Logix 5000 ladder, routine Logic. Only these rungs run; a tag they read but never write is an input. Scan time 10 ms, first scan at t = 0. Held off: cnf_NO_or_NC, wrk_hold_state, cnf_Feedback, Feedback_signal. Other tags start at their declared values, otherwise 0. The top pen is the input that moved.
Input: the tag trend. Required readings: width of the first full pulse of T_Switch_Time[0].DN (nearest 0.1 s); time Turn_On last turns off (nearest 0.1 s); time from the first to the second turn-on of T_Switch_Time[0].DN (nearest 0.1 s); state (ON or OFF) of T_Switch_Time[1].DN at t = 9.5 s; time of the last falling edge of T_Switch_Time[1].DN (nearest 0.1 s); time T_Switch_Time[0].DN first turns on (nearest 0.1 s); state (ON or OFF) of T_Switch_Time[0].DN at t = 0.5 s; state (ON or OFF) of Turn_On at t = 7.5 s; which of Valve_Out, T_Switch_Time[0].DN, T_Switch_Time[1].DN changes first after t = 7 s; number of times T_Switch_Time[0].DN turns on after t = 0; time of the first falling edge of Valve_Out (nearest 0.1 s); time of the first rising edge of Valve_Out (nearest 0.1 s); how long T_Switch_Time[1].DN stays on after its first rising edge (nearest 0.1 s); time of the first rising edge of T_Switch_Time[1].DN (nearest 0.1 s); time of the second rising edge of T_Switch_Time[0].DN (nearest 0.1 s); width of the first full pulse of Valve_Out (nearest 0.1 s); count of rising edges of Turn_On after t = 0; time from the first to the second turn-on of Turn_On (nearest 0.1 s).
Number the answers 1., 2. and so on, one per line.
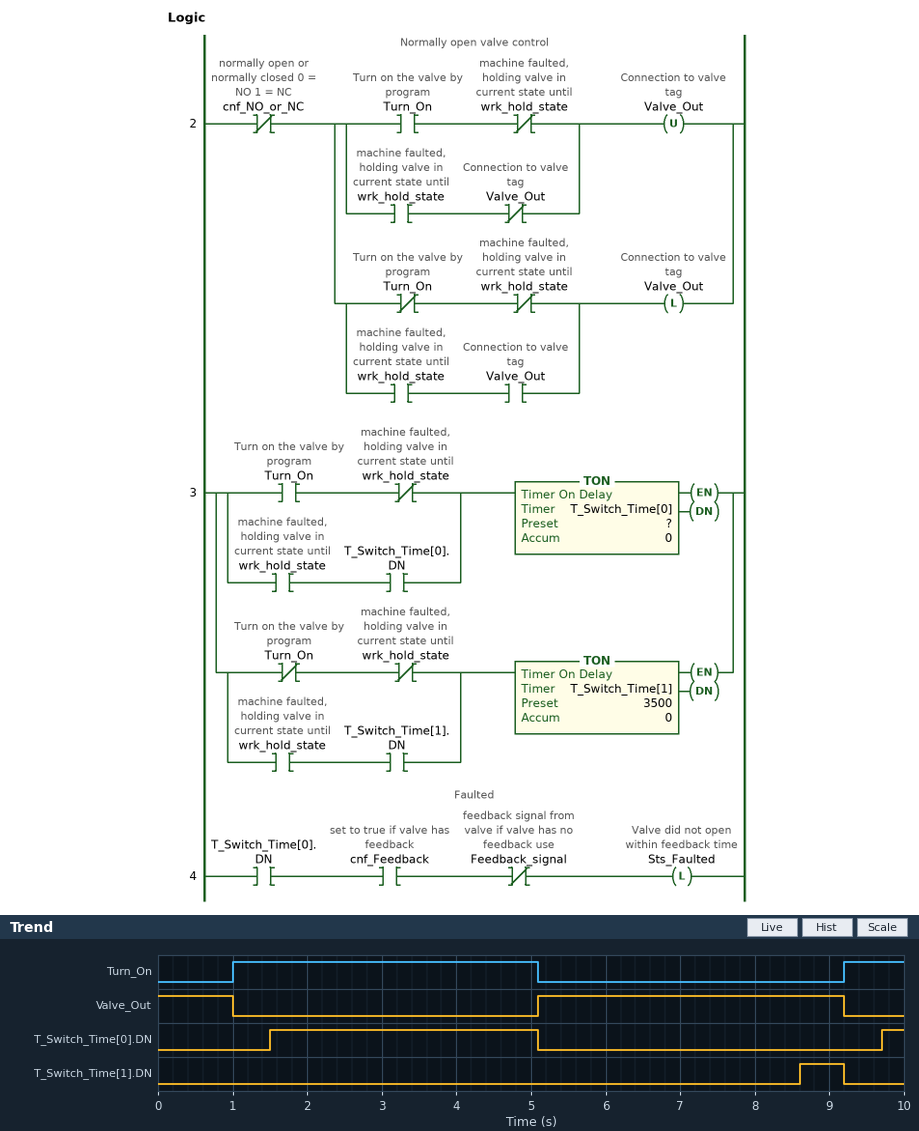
1. 3.6 s
2. 5.1 s
3. 8.2 s
4. OFF
5. 9.2 s
6. 1.5 s
7. OFF
8. OFF
9. T_Switch_Time[1].DN
10. 2
11. 1.0 s
12. 5.1 s
13. 0.6 s
14. 8.6 s
15. 9.7 s
16. 4.1 s
17. 2
18. 8.2 s
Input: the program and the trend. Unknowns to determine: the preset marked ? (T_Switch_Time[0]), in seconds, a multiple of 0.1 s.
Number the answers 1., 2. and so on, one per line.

1. 0.5 s
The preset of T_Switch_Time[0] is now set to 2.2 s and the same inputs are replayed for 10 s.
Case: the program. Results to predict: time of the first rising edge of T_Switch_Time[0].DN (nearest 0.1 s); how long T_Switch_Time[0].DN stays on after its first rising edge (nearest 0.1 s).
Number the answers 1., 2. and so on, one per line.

1. 3.2 s
2. 1.9 s
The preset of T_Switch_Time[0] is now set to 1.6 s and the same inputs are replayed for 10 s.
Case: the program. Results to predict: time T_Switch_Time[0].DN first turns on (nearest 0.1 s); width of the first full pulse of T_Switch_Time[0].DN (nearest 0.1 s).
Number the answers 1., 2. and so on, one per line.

1. 2.6 s
2. 2.5 s
